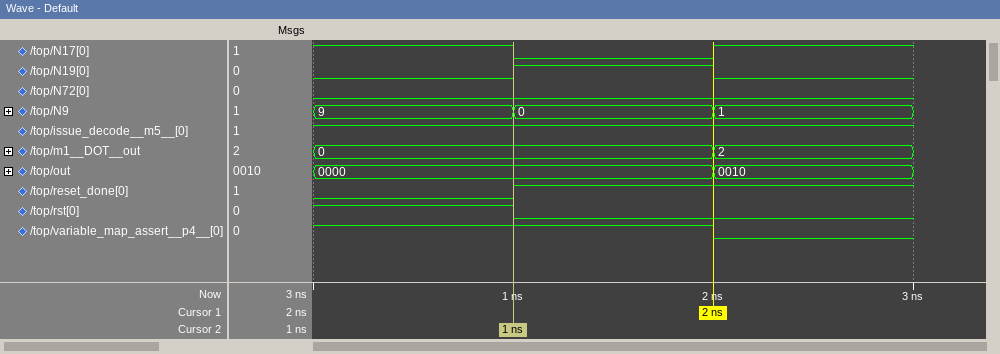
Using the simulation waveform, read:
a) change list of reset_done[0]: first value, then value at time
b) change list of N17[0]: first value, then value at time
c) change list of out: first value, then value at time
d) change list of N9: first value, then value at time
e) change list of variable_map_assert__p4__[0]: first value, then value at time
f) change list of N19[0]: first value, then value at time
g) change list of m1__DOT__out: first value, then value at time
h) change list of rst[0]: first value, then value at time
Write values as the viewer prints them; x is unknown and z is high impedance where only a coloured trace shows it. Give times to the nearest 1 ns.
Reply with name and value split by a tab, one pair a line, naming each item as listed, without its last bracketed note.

change list of reset_done[0]: first value, then value at time	0, 1 at 1 ns
change list of N17[0]: first value, then value at time	1, 0 at 1 ns, 1 at 2 ns
change list of out: first value, then value at time	0000, 0010 at 2 ns
change list of N9: first value, then value at time	9, 0 at 1 ns, 1 at 2 ns
change list of variable_map_assert__p4__[0]: first value, then value at time	1, 0 at 2 ns
change list of N19[0]: first value, then value at time	0, 1 at 1 ns, 0 at 2 ns
change list of m1__DOT__out: first value, then value at time	0, 2 at 2 ns
change list of rst[0]: first value, then value at time	1, 0 at 1 ns
